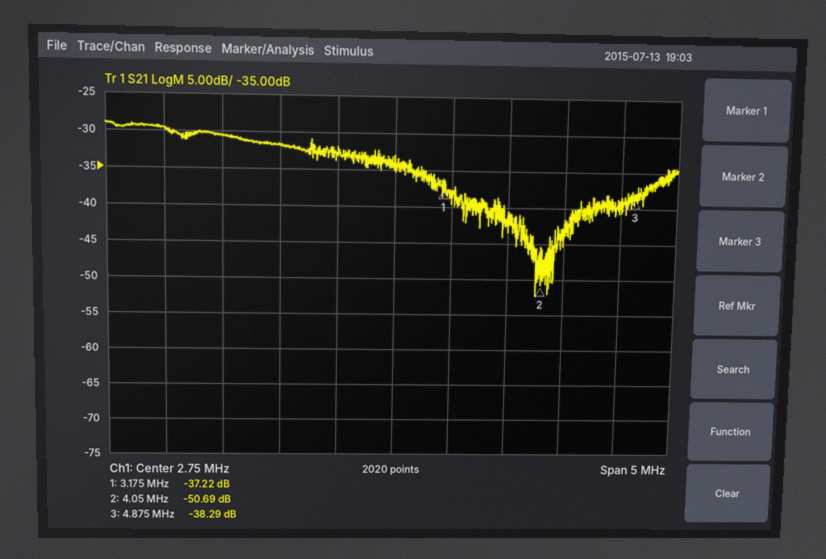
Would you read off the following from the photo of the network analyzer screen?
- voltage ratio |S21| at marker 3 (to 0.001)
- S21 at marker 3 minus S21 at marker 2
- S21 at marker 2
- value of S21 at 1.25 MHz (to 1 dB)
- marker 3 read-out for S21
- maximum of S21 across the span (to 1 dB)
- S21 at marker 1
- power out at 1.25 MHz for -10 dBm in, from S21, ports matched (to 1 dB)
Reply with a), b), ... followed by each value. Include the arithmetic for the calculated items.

a) 10^(-38.29/20) ≈ 0.012
b) -38.29 − (-50.69) = 12.40 dB
c) -50.69 dB
d) -31 dB
e) -38.29 dB
f) -29 dB
g) -37.22 dB
h) -10 dBm + (-31 dB) = -41 dBm
